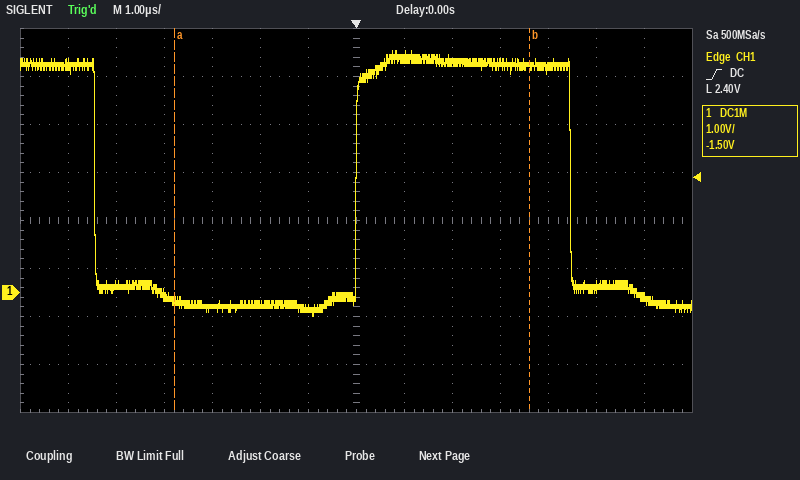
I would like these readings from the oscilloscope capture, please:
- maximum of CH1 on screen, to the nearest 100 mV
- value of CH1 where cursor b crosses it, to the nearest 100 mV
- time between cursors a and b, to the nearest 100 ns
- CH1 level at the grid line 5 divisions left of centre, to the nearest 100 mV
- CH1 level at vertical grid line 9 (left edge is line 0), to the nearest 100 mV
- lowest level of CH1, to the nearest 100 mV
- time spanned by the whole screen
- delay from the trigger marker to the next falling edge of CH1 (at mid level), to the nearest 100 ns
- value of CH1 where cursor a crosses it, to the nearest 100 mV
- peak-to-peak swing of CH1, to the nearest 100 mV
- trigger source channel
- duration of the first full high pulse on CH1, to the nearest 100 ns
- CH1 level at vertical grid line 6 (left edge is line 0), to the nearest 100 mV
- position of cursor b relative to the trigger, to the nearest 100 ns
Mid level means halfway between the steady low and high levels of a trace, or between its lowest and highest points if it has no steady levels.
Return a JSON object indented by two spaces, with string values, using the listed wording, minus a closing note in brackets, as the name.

{
  "maximum of CH1 on screen, to the nearest 100 mV": "5.0 V",
  "value of CH1 where cursor b crosses it, to the nearest 100 mV": "4.7 V",
  "time between cursors a and b, to the nearest 100 ns": "7.4 µs",
  "CH1 level at the grid line 5 divisions left of centre, to the nearest 100 mV": "200 mV",
  "CH1 level at vertical grid line 9 (left edge is line 0), to the nearest 100 mV": "4.8 V",
  "lowest level of CH1, to the nearest 100 mV": "-500 mV",
  "time spanned by the whole screen": "14 µs",
  "delay from the trigger marker to the next falling edge of CH1 (at mid level), to the nearest 100 ns": "4.5 µs",
  "value of CH1 where cursor a crosses it, to the nearest 100 mV": "-200 mV",
  "peak-to-peak swing of CH1, to the nearest 100 mV": "5.5 V",
  "trigger source channel": "CH1",
  "duration of the first full high pulse on CH1, to the nearest 100 ns": "4.5 µs",
  "CH1 level at vertical grid line 6 (left edge is line 0), to the nearest 100 mV": "-300 mV",
  "position of cursor b relative to the trigger, to the nearest 100 ns": "+3.6 µs"
}
